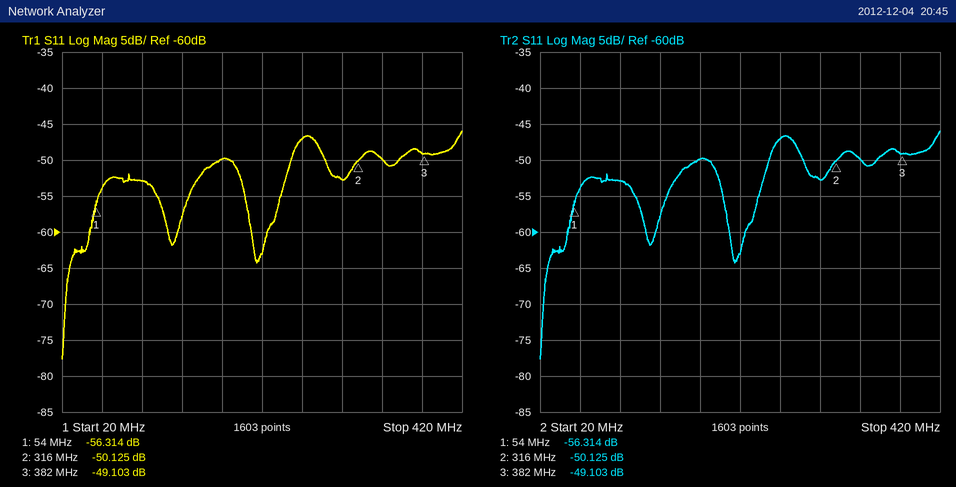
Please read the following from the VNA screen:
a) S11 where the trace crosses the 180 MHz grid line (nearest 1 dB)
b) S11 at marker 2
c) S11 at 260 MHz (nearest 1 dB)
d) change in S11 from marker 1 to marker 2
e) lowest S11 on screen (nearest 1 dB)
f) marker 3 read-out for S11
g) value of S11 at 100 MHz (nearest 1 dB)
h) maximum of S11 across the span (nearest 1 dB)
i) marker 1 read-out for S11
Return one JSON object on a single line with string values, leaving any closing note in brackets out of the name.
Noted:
{"S11 where the trace crosses the 180 MHz grid line": "-50 dB", "S11 at marker 2": "-50.125 dB", "S11 at 260 MHz": "-47 dB", "change in S11 from marker 1 to marker 2": "6.189 dB", "lowest S11 on screen": "-78 dB", "marker 3 read-out for S11": "-49.103 dB", "value of S11 at 100 MHz": "-53 dB", "maximum of S11 across the span": "-46 dB", "marker 1 read-out for S11": "-56.314 dB"}
